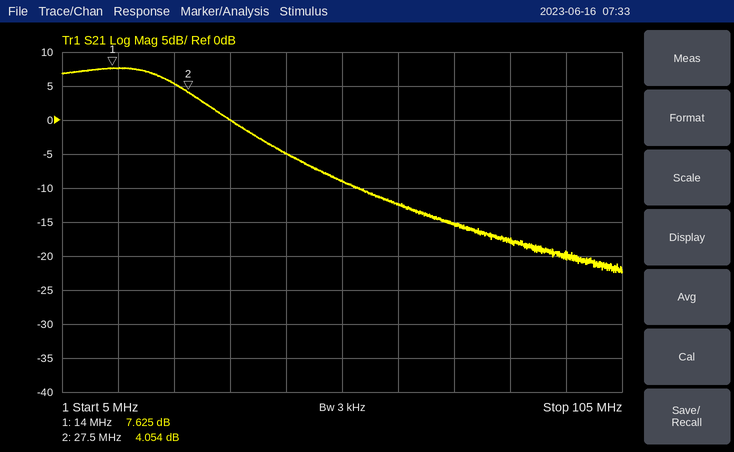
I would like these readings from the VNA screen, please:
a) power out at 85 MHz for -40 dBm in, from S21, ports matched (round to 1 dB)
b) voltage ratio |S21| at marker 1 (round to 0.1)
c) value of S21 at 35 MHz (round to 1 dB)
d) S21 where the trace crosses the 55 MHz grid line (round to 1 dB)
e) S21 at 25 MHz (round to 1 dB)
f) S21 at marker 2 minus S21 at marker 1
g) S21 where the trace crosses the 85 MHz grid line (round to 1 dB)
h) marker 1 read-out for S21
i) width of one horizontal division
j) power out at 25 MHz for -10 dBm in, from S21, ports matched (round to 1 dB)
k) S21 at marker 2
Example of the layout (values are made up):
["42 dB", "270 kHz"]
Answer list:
["-58 dBm", "2.4", "0 dB", "-9 dB", "5 dB", "-3.571 dB", "-18 dB", "7.625 dB", "10 MHz", "-5 dBm", "4.054 dB"]
